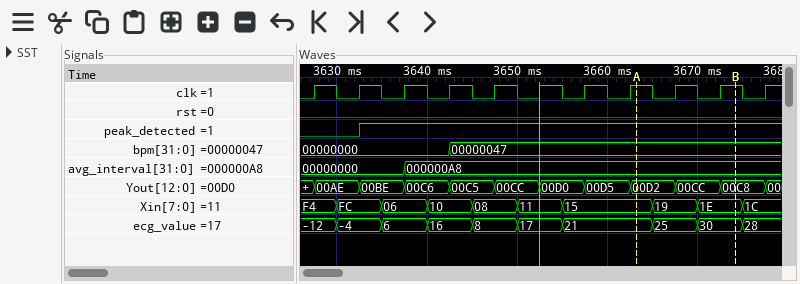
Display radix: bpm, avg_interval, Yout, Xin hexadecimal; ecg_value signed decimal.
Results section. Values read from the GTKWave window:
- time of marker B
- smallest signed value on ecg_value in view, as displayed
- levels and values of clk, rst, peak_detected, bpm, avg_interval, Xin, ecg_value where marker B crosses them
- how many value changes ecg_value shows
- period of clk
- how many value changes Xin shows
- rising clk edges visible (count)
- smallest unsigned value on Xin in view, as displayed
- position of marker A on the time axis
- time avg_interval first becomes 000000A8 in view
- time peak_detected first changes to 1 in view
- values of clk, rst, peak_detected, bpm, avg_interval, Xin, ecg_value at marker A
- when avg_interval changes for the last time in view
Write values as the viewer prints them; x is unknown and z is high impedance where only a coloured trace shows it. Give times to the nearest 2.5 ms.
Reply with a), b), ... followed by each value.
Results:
a) 3675 ms
b) -12
c) clk=1, rst=0, peak_detected=1, bpm=00000047, avg_interval=000000A8, Xin=1E, ecg_value=30
d) 9
e) 5 ms
f) 9
g) 11
h) 06
i) 3662.5 ms
j) 3637.5 ms
k) 3632.5 ms
l) clk=1, rst=0, peak_detected=1, bpm=00000047, avg_interval=000000A8, Xin=15, ecg_value=21
m) 3637.5 ms
